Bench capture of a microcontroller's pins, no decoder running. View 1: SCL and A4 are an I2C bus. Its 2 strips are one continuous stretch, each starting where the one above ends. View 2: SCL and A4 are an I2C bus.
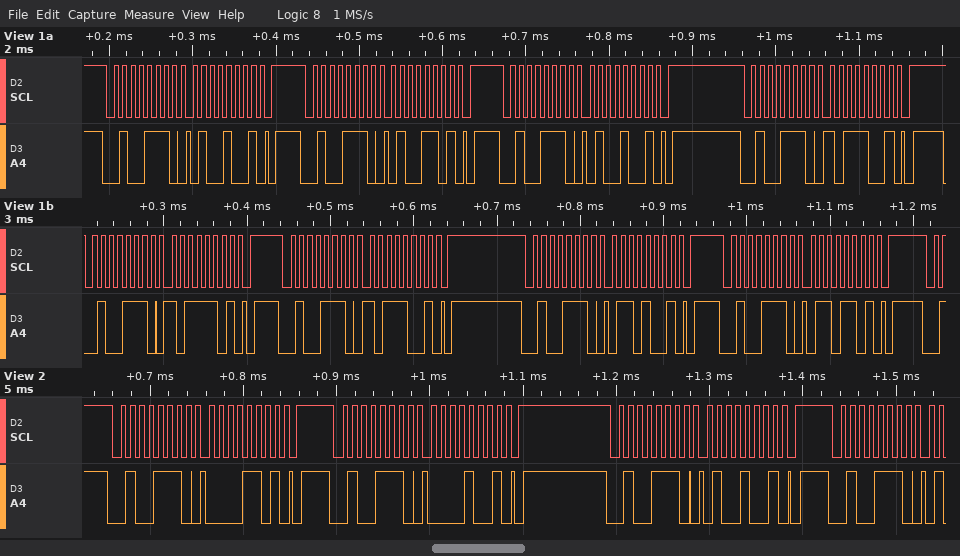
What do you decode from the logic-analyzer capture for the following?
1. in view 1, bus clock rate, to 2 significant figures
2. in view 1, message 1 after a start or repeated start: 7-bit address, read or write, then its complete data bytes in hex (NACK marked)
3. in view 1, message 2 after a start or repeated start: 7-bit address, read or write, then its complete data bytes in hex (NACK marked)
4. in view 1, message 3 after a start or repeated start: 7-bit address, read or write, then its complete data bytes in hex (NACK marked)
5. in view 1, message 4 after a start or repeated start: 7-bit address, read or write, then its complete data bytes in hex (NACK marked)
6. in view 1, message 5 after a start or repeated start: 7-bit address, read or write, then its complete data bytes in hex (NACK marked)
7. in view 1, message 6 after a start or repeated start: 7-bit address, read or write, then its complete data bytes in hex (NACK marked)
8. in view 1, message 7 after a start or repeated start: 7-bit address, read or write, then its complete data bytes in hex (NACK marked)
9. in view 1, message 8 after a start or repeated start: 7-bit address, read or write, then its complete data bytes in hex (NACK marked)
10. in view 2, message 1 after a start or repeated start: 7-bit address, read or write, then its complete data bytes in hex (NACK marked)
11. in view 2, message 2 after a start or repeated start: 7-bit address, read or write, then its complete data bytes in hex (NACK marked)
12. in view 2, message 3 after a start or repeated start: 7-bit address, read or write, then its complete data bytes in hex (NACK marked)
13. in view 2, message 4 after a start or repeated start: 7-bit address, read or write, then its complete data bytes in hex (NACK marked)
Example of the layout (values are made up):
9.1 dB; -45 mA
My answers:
100 kHz; 0x27 write: 49; 0x27 write: 4D; 0x27 write: 49; 0x27 write: B9; 0x27 write: BD; 0x27 write: B9; 0x27 write: 69; 0x27 write: 6D; 0x27 write: 0D; 0x27 write: 09; 0x27 write: 49; 0x27 write
